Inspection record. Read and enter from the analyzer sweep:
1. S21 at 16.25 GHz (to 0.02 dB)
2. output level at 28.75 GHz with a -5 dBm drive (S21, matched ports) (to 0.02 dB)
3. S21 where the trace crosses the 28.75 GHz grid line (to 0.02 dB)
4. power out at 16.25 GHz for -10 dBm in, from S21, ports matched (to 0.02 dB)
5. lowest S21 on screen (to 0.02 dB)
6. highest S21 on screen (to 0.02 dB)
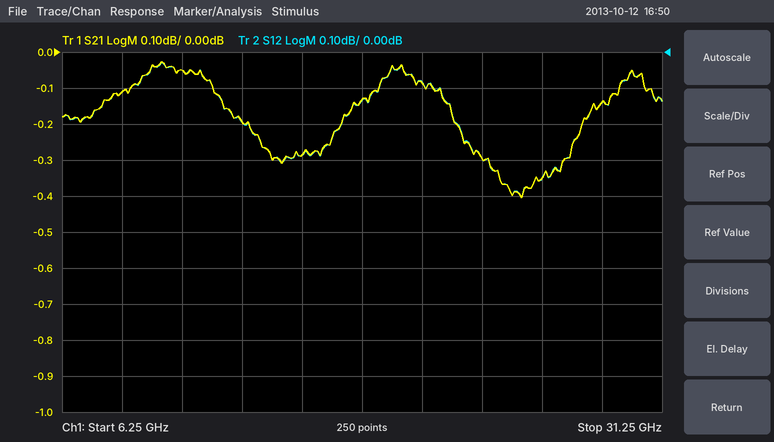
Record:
-0.28 dB
-5.14 dBm
-0.14 dB
-10.28 dBm
-0.40 dB
-0.02 dB
